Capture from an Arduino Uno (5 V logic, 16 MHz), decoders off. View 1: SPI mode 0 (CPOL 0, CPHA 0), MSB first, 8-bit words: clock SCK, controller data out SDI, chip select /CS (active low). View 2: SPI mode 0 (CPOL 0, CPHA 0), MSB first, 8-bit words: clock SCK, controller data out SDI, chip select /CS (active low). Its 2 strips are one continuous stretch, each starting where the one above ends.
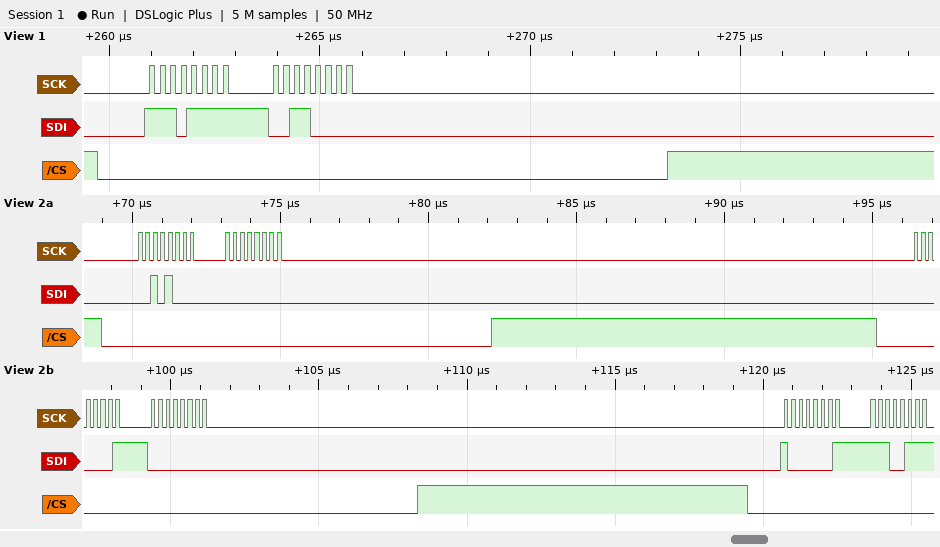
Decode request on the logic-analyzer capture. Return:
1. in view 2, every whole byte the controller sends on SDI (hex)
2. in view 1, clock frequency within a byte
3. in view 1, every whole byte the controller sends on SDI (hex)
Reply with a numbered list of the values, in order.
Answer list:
1. 28 00 01 00 81 E7
2. 4 MHz
3. EF 30
